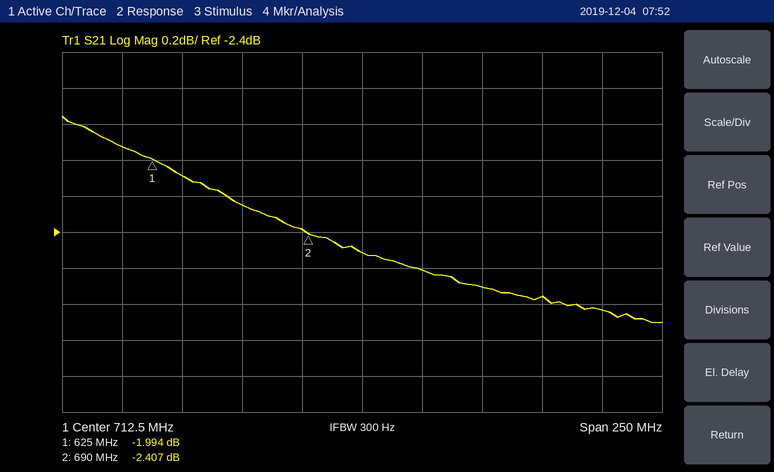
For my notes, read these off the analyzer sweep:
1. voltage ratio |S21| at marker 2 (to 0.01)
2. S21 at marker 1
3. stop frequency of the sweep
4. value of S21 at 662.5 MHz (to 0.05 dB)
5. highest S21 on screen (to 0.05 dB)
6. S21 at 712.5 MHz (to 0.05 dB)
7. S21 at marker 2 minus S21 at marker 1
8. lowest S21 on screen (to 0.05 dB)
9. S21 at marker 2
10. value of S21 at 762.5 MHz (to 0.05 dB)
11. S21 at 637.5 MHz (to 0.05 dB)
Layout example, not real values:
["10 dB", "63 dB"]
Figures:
["0.76", "-1.994 dB", "837.5 MHz", "-2.25 dB", "-1.75 dB", "-2.50 dB", "-0.413 dB", "-2.90 dB", "-2.407 dB", "-2.70 dB", "-2.10 dB"]
